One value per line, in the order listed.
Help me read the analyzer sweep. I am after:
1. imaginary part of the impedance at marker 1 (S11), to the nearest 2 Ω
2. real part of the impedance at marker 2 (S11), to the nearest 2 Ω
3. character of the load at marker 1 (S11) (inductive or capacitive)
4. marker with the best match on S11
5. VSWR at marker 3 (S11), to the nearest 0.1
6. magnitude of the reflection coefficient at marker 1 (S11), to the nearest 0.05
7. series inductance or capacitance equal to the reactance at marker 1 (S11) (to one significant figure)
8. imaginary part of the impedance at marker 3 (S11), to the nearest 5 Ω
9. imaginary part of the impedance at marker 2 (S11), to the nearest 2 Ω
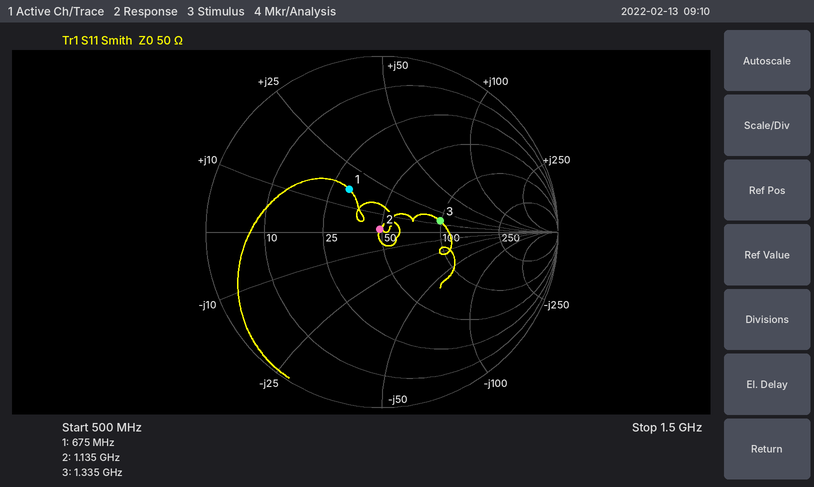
+16 Ω
48 Ω
inductive
marker 2
2.0
0.30
4 nH
+15 Ω
+2 Ω
